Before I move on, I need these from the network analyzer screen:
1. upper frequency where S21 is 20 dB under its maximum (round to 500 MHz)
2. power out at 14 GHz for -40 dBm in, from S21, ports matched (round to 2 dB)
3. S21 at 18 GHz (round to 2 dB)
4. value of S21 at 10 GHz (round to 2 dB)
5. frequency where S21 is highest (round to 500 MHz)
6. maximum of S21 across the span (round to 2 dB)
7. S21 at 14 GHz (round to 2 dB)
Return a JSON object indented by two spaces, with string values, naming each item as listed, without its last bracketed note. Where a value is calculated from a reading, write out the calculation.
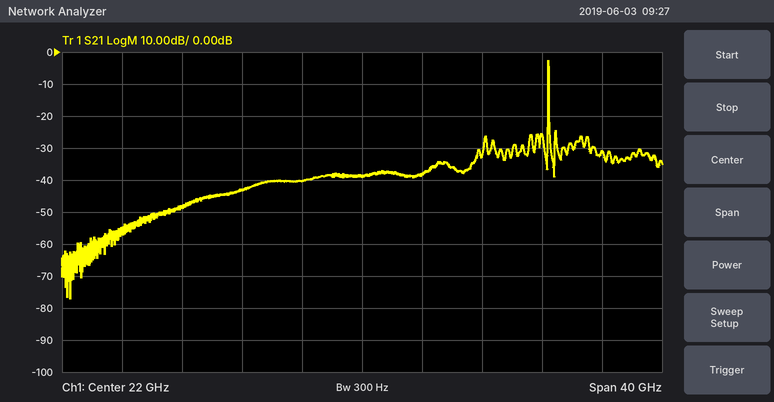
{
  "upper frequency where S21 is 20 dB under its maximum": "34.5 GHz",
  "power out at 14 GHz for -40 dBm in, from S21, ports matched": "-40 dBm + (-44 dB) = -84 dBm",
  "S21 at 18 GHz": "-40 dB",
  "value of S21 at 10 GHz": "-48 dB",
  "frequency where S21 is highest": "34.5 GHz",
  "maximum of S21 across the span": "-2 dB",
  "S21 at 14 GHz": "-44 dB"
}
